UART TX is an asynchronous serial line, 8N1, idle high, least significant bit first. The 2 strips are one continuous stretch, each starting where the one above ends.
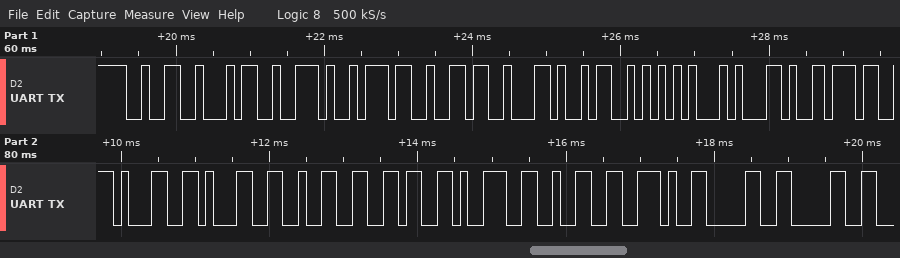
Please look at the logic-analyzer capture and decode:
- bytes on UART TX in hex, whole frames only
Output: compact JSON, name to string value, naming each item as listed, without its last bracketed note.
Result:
{"bytes on UART TX in hex, whole frames only": "0x32 0x34 0x2E 0x37 0x36 0x2C 0x53 0x45 0x2C 0x37 0x31 0x31 0x32 0x36 0x39 0x32 0x2E 0x30 0x30"}
